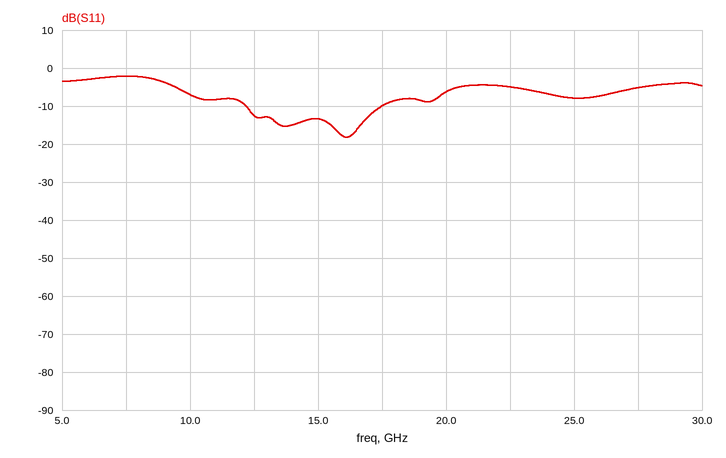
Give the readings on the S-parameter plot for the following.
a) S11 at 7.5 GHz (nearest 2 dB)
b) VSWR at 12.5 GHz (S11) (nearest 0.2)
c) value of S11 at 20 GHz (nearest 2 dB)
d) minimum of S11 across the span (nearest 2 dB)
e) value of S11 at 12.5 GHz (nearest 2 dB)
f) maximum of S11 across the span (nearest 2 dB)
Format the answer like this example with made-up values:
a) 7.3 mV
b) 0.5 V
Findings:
a) -2 dB
b) 1.6
c) -6 dB
d) -18 dB
e) -12 dB
f) -2 dB
